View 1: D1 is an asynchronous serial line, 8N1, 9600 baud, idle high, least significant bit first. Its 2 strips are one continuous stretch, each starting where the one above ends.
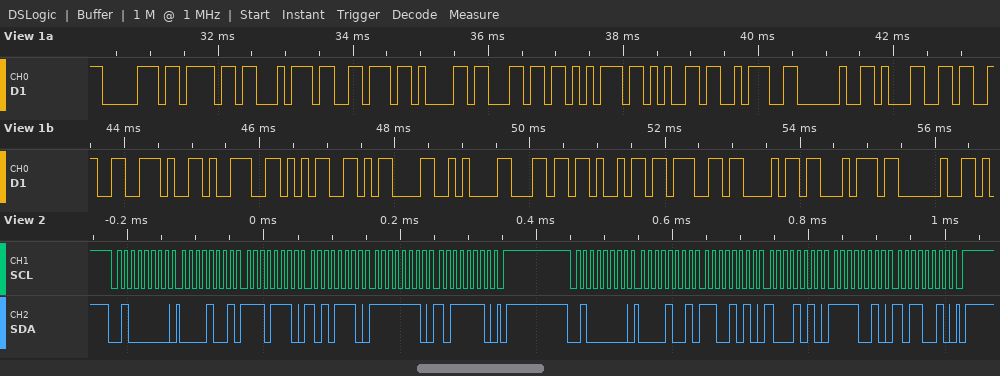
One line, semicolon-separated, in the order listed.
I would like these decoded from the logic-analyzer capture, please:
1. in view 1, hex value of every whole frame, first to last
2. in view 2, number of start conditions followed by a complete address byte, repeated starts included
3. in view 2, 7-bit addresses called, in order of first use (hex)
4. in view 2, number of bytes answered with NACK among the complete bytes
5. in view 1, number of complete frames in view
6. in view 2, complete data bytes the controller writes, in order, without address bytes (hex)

70 6F 74 76 61 6C 75 65 3A 20 31 33 2E 39 35 0D 0A 6C 69 67 68 74 20; 2; 0x20; 0; 23; 09 EE AE FE BE 09 CA 8A F2 B2
